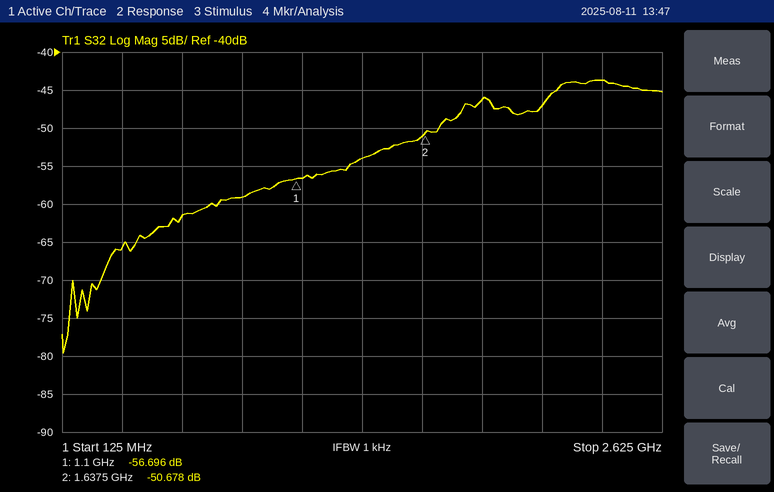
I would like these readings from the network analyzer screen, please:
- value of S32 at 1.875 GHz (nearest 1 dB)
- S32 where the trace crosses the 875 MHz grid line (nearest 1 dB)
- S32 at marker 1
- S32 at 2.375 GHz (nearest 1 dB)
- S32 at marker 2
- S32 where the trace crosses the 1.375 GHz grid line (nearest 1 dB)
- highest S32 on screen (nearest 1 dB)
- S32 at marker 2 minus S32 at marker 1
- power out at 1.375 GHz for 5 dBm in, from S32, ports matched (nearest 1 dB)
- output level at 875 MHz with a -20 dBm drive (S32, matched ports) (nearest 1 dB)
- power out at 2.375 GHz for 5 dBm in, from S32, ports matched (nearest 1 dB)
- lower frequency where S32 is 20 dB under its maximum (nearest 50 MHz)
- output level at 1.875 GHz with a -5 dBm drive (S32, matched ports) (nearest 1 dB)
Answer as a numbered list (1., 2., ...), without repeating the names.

1. -46 dB
2. -59 dB
3. -56.696 dB
4. -44 dB
5. -50.678 dB
6. -54 dB
7. -44 dB
8. 6.018 dB
9. -49 dBm
10. -79 dBm
11. -39 dBm
12. 500 MHz
13. -51 dBm
